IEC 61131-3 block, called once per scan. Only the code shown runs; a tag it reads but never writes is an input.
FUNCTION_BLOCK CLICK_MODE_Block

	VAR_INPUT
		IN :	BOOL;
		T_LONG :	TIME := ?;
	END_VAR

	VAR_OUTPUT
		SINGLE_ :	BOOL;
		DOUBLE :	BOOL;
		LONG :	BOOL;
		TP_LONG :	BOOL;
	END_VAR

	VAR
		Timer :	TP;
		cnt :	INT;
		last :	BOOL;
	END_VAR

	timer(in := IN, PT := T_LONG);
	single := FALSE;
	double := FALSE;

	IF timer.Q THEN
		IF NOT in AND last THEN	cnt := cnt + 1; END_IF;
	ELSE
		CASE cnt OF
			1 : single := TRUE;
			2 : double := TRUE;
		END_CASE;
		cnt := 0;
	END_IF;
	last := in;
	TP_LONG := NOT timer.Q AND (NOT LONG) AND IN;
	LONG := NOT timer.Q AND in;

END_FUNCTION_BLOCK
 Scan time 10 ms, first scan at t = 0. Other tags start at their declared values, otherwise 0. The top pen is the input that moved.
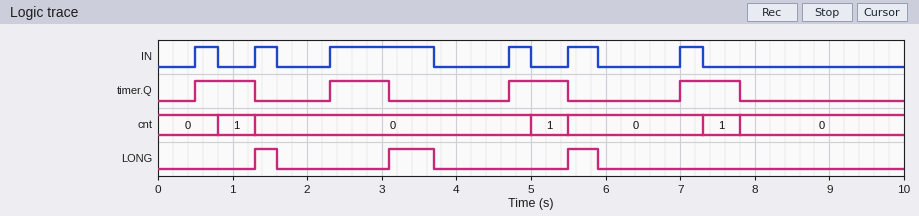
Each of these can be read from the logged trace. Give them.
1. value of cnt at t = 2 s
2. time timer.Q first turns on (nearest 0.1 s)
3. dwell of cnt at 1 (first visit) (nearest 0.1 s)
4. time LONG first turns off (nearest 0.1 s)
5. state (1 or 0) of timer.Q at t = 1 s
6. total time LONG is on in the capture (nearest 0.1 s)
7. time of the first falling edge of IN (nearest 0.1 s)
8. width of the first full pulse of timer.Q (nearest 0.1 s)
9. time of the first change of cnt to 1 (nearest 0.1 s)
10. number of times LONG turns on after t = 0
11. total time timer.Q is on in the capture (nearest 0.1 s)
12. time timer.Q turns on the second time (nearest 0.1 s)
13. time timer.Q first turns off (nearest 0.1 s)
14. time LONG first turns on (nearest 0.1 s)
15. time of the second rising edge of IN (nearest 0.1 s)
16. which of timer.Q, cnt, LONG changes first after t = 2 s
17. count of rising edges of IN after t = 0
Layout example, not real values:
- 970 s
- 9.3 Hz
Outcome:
- 0
- 0.5 s
- 0.5 s
- 1.6 s
- 1
- 1.3 s
- 0.8 s
- 0.8 s
- 0.8 s
- 3
- 3.2 s
- 2.3 s
- 1.3 s
- 1.3 s
- 1.3 s
- timer.Q
- 6
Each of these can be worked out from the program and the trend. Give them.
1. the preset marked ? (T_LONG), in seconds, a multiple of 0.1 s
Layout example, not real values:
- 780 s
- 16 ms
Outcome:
- 0.8 s
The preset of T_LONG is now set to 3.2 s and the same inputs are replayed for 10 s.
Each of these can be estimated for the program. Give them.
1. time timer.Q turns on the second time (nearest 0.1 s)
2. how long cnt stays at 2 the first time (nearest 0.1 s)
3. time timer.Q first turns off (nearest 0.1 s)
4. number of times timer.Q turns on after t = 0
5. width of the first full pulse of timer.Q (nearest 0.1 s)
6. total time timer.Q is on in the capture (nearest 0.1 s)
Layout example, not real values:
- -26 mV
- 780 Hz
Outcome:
- 4.7 s
- 2.1 s
- 3.7 s
- 2
- 3.2 s
- 6.4 s
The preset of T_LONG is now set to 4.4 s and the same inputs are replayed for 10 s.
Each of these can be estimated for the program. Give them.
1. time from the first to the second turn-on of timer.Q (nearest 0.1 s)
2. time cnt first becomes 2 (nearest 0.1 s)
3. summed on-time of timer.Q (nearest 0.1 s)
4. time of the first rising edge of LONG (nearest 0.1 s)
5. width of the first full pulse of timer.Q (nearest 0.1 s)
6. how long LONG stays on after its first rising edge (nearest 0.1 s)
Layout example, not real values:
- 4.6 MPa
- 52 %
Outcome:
- 5.0 s
- 1.6 s
- 8.8 s
- 4.9 s
- 4.4 s
- 0.1 s
